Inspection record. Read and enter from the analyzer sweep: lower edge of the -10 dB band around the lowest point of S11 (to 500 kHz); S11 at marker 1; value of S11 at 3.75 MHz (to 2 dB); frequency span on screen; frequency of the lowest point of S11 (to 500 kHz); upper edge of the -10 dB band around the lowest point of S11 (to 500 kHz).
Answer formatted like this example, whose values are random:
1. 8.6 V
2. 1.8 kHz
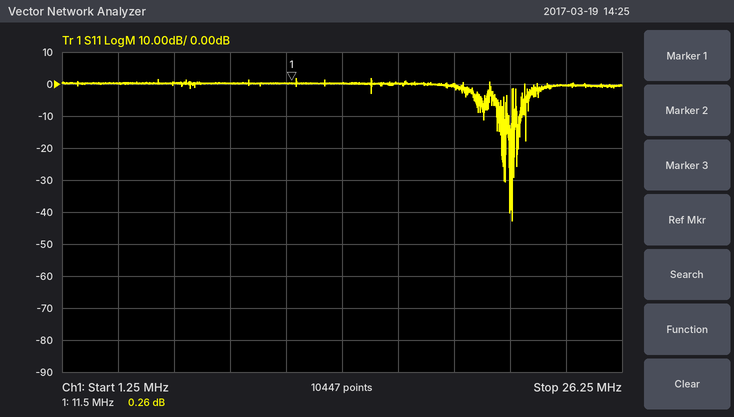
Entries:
1. 21.0 MHz
2. 0.26 dB
3. 0 dB
4. 25 MHz
5. 21.5 MHz
6. 21.5 MHz
